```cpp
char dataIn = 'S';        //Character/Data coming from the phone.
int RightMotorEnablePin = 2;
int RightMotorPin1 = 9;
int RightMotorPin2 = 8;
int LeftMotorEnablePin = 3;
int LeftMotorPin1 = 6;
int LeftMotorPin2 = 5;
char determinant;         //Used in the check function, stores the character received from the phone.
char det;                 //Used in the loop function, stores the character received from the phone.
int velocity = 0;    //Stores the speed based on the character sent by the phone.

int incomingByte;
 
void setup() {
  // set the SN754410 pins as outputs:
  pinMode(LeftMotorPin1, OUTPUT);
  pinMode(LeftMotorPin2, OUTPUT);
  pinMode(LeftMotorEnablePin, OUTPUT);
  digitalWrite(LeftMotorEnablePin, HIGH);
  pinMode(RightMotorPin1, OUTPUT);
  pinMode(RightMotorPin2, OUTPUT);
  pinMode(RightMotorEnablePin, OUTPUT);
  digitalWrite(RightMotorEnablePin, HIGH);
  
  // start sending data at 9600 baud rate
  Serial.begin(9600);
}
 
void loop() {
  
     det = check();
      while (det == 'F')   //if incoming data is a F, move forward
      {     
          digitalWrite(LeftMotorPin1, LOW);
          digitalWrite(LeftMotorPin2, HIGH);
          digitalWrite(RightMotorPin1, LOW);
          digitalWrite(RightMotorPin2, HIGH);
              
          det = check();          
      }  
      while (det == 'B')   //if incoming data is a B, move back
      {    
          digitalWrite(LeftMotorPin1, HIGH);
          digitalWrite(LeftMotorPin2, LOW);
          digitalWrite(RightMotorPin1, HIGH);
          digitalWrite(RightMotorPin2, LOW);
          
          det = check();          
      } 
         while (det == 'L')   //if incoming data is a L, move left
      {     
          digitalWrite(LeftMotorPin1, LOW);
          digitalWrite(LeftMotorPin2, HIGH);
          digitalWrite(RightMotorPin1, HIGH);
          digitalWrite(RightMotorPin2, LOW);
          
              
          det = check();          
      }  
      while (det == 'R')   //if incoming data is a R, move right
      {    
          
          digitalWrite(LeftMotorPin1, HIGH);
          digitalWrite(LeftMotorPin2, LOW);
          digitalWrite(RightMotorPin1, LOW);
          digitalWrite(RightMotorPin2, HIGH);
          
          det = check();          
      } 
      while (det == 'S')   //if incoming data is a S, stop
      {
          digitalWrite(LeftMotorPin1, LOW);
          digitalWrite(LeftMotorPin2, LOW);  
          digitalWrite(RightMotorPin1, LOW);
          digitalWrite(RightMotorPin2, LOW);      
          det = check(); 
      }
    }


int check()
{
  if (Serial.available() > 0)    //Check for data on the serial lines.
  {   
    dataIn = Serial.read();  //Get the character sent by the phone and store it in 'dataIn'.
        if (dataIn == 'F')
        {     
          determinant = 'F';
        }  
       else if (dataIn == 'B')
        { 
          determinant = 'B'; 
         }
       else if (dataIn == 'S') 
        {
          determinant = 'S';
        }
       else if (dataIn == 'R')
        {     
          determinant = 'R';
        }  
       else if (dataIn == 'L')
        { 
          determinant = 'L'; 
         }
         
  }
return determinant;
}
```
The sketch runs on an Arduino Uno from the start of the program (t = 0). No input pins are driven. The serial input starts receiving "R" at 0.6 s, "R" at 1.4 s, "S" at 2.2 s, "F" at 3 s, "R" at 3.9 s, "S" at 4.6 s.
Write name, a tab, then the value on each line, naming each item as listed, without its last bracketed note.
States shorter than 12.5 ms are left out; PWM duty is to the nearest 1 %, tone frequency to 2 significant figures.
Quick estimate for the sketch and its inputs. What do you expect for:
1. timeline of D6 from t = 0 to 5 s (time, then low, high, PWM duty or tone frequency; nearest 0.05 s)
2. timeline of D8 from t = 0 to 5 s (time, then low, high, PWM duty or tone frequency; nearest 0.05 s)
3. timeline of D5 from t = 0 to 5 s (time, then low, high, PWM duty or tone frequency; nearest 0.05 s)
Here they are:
timeline of D6 from t = 0 to 5 s	0 s low; 0.6 s high; 2.2 s low; 3.9 s high; 4.6 s low
timeline of D8 from t = 0 to 5 s	0 s low; 0.6 s high; 2.2 s low; 3 s high; 4.6 s low
timeline of D5 from t = 0 to 5 s	0 s low; 3 s high; 3.9 s low
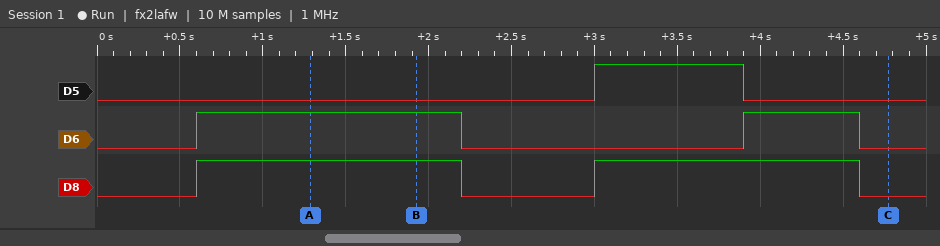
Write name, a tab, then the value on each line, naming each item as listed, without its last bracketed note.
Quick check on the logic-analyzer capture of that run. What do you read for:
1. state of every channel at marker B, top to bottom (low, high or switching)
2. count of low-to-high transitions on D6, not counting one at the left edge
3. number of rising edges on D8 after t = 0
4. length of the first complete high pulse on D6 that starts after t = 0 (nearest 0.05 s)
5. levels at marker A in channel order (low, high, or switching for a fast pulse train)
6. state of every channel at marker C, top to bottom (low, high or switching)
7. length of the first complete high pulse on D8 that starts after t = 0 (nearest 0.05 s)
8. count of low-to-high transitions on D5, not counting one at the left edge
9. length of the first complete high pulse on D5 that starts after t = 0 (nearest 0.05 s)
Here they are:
state of every channel at marker B, top to bottom	D5 low, D6 high, D8 high
count of low-to-high transitions on D6, not counting one at the left edge	2
number of rising edges on D8 after t = 0	2
length of the first complete high pulse on D6 that starts after t = 0	1.60 s
levels at marker A in channel order	D5 low, D6 high, D8 high
state of every channel at marker C, top to bottom	D5 low, D6 low, D8 low
length of the first complete high pulse on D8 that starts after t = 0	1.60 s
count of low-to-high transitions on D5, not counting one at the left edge	1
length of the first complete high pulse on D5 that starts after t = 0	0.90 s
